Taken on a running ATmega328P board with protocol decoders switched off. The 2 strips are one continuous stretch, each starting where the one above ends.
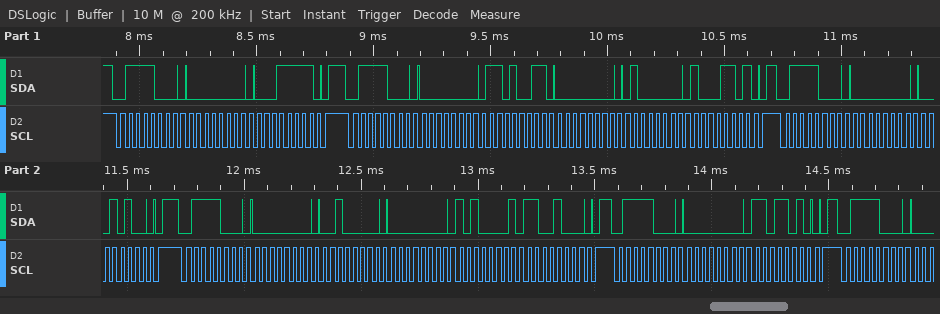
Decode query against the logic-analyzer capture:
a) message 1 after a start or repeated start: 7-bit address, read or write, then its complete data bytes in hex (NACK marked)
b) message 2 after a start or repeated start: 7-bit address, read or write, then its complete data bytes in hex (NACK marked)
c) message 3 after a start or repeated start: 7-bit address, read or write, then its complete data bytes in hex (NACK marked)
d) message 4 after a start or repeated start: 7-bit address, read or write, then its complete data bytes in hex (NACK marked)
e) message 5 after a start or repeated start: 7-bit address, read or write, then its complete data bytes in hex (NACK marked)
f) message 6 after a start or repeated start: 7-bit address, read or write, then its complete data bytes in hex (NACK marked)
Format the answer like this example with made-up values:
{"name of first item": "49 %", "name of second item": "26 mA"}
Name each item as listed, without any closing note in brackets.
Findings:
{"message 1 after a start or repeated start: 7-bit address, read or write, then its complete data bytes in hex": "0x3C write: 00 1F", "message 2 after a start or repeated start: 7-bit address, read or write, then its complete data bytes in hex": "0x3C write: 00 D3 00 40 8D", "message 3 after a start or repeated start: 7-bit address, read or write, then its complete data bytes in hex": "0x3C write: 00 14", "message 4 after a start or repeated start: 7-bit address, read or write, then its complete data bytes in hex": "0x3C write: 00 20 00 A1 C8", "message 5 after a start or repeated start: 7-bit address, read or write, then its complete data bytes in hex": "0x3C write: 00 DA", "message 6 after a start or repeated start: 7-bit address, read or write, then its complete data bytes in hex": "0x3C write"}
